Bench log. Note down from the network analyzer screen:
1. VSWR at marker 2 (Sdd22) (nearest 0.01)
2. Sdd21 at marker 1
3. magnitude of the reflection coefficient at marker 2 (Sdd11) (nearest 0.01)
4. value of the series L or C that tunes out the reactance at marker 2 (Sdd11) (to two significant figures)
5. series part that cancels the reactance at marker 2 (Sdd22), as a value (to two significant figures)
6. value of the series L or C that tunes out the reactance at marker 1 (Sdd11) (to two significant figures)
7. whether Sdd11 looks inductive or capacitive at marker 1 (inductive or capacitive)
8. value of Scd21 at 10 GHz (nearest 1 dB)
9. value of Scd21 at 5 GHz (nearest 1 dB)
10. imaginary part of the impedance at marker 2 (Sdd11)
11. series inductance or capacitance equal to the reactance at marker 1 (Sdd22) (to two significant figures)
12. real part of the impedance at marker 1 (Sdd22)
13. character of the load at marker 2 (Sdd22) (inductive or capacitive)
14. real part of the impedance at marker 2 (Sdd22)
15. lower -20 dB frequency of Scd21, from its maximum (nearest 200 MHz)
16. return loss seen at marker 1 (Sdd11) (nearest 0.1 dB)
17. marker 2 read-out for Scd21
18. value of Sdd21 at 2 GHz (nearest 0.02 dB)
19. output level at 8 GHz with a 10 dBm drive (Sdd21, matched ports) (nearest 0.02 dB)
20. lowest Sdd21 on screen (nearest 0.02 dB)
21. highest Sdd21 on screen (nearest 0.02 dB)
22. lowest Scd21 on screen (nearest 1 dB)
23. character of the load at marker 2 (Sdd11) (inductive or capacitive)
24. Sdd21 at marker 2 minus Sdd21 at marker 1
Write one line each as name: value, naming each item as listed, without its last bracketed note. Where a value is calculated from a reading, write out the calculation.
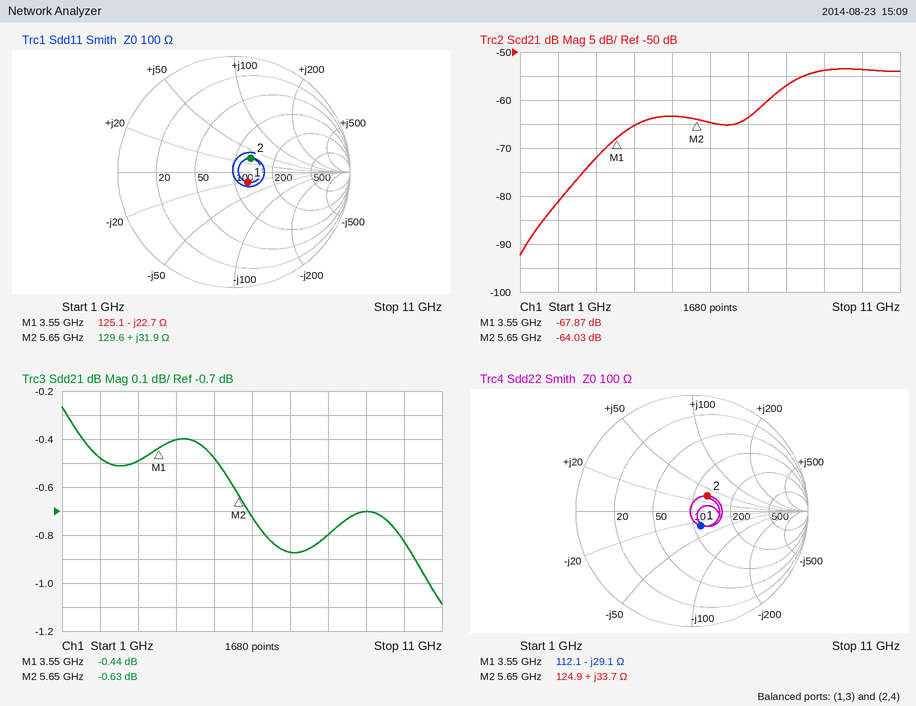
VSWR at marker 2 (Sdd22): 1.45
Sdd21 at marker 1: -0.44 dB
magnitude of the reflection coefficient at marker 2 (Sdd11): 0.19
value of the series L or C that tunes out the reactance at marker 2 (Sdd11): C = 1/(2π × 5.65 GHz × 31.9 Ω) ≈ 883 fF, so 880 fF to two significant figures
series part that cancels the reactance at marker 2 (Sdd22), as a value: C = 1/(2π × 5.65 GHz × 33.7 Ω) ≈ 836 fF, so 840 fF to two significant figures
value of the series L or C that tunes out the reactance at marker 1 (Sdd11): L = 22.7 Ω/(2π × 3.55 GHz) ≈ 1.0 nH
whether Sdd11 looks inductive or capacitive at marker 1: capacitive
value of Scd21 at 10 GHz: -54 dB
value of Scd21 at 5 GHz: -63 dB
imaginary part of the impedance at marker 2: +31.9 Ω
series inductance or capacitance equal to the reactance at marker 1 (Sdd22): C = 1/(2π × 3.55 GHz × 29.1 Ω) ≈ 1.5 pF
real part of the impedance at marker 1: 112.1 Ω
character of the load at marker 2 (Sdd22): inductive
real part of the impedance at marker 2: 124.9 Ω
lower -20 dB frequency of Scd21, from its maximum: 2.8 GHz
return loss seen at marker 1 (Sdd11): 16.5 dB
marker 2 read-out for Scd21: -64.03 dB
value of Sdd21 at 2 GHz: -0.48 dB
output level at 8 GHz with a 10 dBm drive (Sdd21, matched ports): 10 dBm + (-0.80 dB) = 9.20 dBm
lowest Sdd21 on screen: -1.08 dB
highest Sdd21 on screen: -0.26 dB
lowest Scd21 on screen: -92 dB
character of the load at marker 2 (Sdd11): inductive
Sdd21 at marker 2 minus Sdd21 at marker 1: -0.63 − (-0.44) = -0.19 dB
